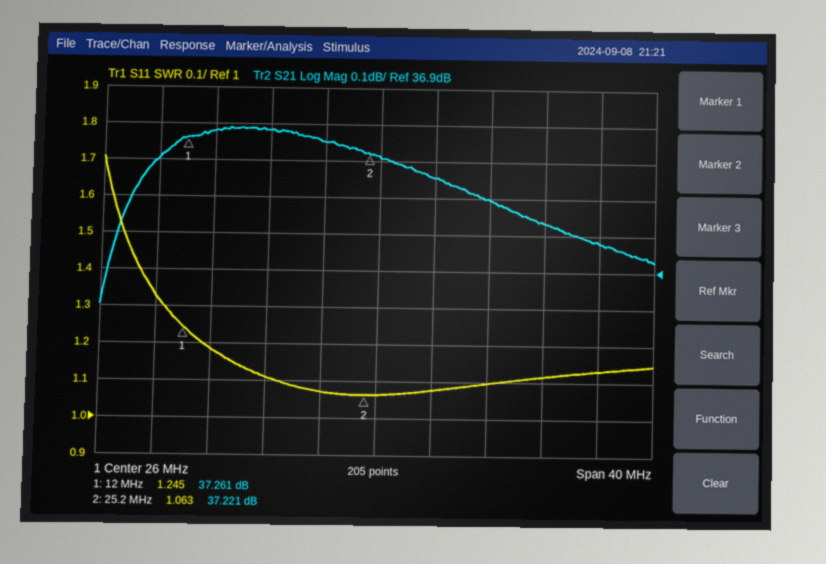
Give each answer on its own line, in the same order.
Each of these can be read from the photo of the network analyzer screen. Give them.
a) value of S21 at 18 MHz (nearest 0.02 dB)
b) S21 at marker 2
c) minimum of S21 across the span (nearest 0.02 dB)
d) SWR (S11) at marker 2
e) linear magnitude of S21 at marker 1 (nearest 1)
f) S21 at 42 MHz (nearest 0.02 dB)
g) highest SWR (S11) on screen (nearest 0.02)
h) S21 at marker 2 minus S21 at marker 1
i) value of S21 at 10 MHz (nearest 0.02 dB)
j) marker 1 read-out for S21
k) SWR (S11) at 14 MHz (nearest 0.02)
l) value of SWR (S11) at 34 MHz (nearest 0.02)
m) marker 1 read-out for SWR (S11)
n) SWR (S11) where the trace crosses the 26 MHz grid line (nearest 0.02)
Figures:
37.28 dB
37.221 dB
36.80 dB
1.063
73
36.98 dB
1.70
-0.040 dB
37.20 dB
37.261 dB
1.18
1.10
1.245
1.06
